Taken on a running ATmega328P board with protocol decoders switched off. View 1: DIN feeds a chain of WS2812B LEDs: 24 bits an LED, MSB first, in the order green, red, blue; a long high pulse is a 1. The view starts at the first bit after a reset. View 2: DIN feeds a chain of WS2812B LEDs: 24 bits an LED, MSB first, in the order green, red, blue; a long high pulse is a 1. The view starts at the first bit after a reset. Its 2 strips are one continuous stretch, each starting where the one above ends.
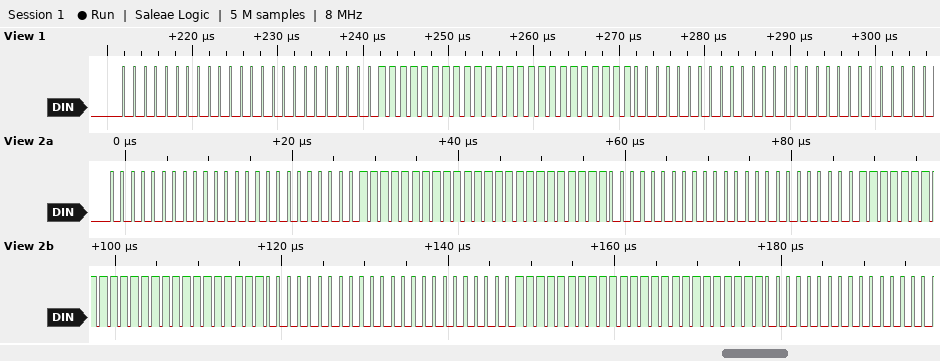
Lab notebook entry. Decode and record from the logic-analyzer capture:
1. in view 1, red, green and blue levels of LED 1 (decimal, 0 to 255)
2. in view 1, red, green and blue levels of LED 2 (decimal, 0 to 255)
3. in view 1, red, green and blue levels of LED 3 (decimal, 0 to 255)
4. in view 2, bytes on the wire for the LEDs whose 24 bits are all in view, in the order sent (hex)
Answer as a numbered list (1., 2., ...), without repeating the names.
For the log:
1. 0, 0, 0
2. 255, 255, 255
3. 0, 0, 0
4. 00 00 00 FF FF FF 00 00 00 FF FF FF 00 00 00 FF FF FF
